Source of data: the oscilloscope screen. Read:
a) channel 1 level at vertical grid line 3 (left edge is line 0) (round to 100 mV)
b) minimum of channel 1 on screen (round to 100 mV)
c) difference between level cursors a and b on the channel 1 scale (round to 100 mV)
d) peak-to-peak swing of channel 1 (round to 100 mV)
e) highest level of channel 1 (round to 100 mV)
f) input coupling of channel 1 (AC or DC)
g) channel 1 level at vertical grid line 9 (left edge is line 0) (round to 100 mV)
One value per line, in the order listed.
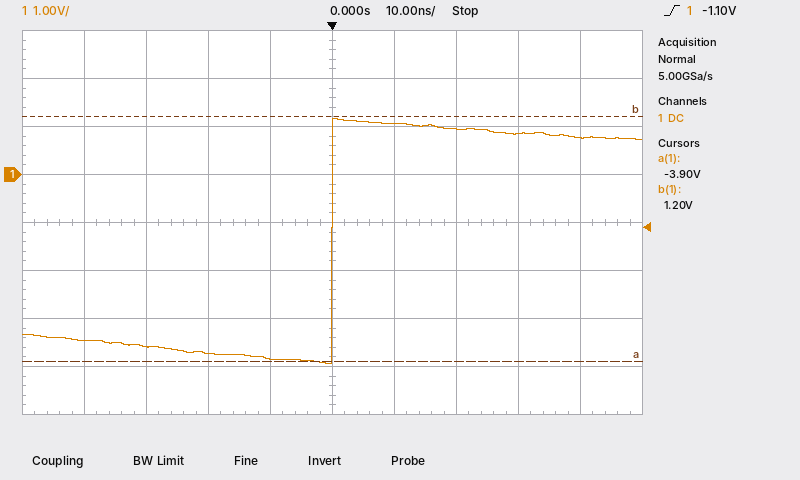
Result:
-3.7 V
-3.9 V
5.1 V
5.1 V
1.2 V
DC
800 mV
